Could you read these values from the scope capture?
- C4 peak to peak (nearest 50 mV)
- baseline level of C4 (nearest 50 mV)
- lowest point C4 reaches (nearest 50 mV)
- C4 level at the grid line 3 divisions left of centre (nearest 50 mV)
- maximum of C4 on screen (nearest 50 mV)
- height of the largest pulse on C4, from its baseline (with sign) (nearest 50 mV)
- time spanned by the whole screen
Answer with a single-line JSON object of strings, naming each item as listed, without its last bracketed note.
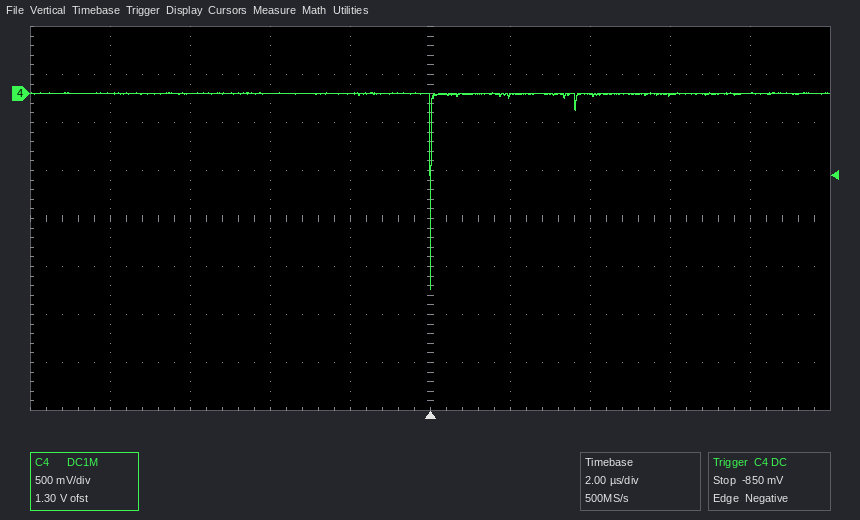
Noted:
{"C4 peak to peak": "2.05 V", "baseline level of C4": "0 mV", "lowest point C4 reaches": "-2.05 V", "C4 level at the grid line 3 divisions left of centre": "0 mV", "maximum of C4 on screen": "0 mV", "height of the largest pulse on C4, from its baseline (with sign)": "-2.05 V", "time spanned by the whole screen": "20 µs"}
